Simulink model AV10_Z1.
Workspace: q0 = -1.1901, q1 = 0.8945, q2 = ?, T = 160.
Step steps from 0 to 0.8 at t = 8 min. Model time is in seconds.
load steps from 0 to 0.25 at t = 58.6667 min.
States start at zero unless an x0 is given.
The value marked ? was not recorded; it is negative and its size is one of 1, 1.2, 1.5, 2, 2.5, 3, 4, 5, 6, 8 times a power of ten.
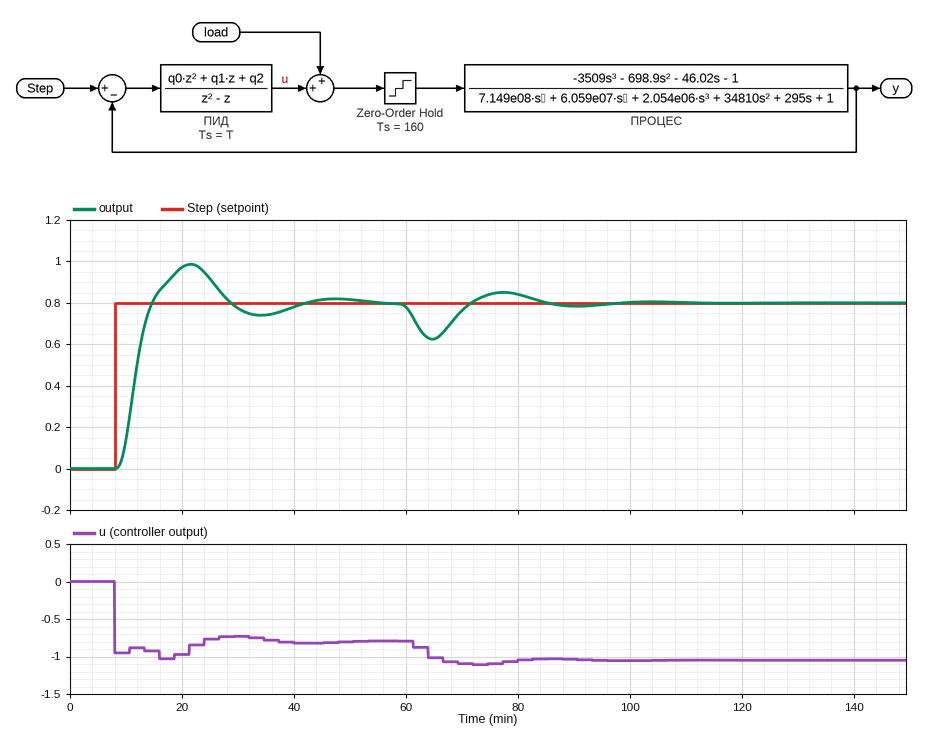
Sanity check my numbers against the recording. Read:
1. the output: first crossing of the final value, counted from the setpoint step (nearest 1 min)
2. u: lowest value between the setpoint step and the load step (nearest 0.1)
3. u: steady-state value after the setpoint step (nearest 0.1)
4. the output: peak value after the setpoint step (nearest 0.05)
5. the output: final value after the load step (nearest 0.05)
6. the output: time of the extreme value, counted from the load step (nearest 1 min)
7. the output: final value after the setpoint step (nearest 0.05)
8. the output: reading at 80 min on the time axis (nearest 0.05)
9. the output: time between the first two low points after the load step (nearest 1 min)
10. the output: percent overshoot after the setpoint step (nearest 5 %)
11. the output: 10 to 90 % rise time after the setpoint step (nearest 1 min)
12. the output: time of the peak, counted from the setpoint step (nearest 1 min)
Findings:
7 min
-1.0
-0.8
1.00
0.80
6 min
0.80
0.85
26 min
25 %
4 min
14 min
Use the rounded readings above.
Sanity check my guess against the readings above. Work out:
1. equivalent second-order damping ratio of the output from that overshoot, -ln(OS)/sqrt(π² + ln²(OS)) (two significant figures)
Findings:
0.40
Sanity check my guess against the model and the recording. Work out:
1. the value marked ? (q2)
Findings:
-0.5
